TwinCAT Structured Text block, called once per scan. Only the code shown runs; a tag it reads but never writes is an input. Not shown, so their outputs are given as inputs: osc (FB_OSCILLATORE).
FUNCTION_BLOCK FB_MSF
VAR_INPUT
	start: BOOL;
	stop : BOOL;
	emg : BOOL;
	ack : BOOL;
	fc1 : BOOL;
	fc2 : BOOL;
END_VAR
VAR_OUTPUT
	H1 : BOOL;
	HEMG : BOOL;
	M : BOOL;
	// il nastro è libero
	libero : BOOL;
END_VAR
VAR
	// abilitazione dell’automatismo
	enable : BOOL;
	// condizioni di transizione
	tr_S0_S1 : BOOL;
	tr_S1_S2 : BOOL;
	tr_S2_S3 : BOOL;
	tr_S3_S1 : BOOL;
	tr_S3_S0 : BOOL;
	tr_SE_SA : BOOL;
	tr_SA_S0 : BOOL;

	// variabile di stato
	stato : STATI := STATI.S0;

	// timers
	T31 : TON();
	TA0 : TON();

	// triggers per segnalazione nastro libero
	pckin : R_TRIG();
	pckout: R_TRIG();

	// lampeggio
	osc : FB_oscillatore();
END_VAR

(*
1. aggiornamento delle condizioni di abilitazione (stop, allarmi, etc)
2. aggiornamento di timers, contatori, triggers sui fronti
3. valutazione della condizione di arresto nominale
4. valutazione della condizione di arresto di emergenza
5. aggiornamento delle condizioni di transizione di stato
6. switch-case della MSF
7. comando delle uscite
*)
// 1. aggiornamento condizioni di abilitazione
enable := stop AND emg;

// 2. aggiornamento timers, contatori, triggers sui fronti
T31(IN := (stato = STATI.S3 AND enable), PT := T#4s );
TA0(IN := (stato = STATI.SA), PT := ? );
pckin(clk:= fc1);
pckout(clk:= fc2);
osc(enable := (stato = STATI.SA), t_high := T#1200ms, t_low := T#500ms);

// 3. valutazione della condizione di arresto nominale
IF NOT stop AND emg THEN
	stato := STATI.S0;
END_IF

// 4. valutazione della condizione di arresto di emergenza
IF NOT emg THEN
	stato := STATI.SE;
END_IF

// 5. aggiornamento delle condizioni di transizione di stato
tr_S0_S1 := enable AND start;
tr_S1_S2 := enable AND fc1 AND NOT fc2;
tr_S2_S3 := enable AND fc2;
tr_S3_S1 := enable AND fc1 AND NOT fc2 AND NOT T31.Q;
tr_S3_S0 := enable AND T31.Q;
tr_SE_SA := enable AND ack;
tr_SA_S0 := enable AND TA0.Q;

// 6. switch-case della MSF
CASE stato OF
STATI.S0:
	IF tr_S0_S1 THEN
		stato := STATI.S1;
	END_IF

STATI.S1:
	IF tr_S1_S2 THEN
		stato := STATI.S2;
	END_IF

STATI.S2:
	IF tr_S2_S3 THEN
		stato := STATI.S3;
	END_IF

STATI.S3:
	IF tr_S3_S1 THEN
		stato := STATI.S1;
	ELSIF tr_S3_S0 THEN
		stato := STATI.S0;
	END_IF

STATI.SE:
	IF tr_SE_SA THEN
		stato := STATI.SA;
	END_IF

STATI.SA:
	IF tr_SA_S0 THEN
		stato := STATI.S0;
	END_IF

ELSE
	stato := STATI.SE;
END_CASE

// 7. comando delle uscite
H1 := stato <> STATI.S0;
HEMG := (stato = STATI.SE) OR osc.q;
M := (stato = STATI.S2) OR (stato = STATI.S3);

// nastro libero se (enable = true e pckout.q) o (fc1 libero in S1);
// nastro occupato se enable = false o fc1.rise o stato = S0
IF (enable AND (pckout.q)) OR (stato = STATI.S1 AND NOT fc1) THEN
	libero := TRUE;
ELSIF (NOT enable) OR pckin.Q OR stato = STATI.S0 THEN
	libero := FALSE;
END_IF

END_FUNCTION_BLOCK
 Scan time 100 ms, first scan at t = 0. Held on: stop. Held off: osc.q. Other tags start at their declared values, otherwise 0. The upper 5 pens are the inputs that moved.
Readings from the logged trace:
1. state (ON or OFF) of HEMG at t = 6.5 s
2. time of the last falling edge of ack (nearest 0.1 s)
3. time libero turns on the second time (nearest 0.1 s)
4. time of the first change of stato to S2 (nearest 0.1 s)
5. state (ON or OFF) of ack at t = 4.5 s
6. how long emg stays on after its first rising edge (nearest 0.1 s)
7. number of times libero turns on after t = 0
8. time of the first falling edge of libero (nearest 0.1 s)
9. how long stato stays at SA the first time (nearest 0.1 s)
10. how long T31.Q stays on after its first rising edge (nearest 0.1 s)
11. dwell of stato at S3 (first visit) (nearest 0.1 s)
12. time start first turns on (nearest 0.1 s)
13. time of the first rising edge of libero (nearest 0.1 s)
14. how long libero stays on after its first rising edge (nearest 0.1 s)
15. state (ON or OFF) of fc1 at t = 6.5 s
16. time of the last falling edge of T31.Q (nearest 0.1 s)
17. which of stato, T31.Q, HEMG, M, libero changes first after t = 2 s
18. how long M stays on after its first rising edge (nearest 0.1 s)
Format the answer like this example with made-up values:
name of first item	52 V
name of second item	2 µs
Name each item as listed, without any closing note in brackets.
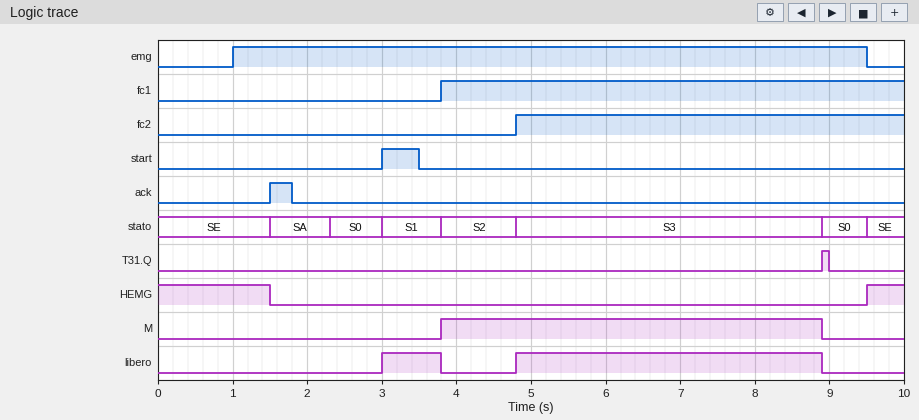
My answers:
state (ON or OFF) of HEMG at t = 6.5 s	OFF
time of the last falling edge of ack	1.8 s
time libero turns on the second time	4.8 s
time of the first change of stato to S2	3.8 s
state (ON or OFF) of ack at t = 4.5 s	OFF
how long emg stays on after its first rising edge	8.5 s
number of times libero turns on after t = 0	2
time of the first falling edge of libero	3.8 s
how long stato stays at SA the first time	0.8 s
how long T31.Q stays on after its first rising edge	0.1 s
dwell of stato at S3 (first visit)	4.1 s
time start first turns on	3.0 s
time of the first rising edge of libero	3.0 s
how long libero stays on after its first rising edge	0.8 s
state (ON or OFF) of fc1 at t = 6.5 s	ON
time of the last falling edge of T31.Q	9.0 s
which of stato, T31.Q, HEMG, M, libero changes first after t = 2 s	stato
how long M stays on after its first rising edge	5.1 s
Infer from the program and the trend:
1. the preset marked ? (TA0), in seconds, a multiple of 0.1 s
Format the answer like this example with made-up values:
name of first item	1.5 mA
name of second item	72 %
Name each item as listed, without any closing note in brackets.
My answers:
the preset marked ? (TA0), in seconds, a multiple of 0.1 s	0.7 s
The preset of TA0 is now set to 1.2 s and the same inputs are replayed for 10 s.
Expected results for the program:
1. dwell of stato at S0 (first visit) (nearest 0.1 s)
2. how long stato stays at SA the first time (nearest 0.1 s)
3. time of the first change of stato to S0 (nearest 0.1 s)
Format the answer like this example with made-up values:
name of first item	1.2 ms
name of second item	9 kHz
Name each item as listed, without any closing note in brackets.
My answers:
dwell of stato at S0 (first visit)	0.2 s
how long stato stays at SA the first time	1.3 s
time of the first change of stato to S0	2.8 s
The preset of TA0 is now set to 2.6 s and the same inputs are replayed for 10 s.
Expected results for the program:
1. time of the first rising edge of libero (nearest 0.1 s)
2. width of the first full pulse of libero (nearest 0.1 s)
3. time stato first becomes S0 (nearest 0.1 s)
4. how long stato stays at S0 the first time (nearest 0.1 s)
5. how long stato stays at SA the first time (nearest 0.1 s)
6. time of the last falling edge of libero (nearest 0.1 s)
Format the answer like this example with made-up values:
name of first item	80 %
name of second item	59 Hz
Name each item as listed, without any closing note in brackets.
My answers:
time of the first rising edge of libero	4.8 s
width of the first full pulse of libero	0.1 s
time stato first becomes S0	4.2 s
how long stato stays at S0 the first time	5.3 s
how long stato stays at SA the first time	2.7 s
time of the last falling edge of libero	4.9 s
